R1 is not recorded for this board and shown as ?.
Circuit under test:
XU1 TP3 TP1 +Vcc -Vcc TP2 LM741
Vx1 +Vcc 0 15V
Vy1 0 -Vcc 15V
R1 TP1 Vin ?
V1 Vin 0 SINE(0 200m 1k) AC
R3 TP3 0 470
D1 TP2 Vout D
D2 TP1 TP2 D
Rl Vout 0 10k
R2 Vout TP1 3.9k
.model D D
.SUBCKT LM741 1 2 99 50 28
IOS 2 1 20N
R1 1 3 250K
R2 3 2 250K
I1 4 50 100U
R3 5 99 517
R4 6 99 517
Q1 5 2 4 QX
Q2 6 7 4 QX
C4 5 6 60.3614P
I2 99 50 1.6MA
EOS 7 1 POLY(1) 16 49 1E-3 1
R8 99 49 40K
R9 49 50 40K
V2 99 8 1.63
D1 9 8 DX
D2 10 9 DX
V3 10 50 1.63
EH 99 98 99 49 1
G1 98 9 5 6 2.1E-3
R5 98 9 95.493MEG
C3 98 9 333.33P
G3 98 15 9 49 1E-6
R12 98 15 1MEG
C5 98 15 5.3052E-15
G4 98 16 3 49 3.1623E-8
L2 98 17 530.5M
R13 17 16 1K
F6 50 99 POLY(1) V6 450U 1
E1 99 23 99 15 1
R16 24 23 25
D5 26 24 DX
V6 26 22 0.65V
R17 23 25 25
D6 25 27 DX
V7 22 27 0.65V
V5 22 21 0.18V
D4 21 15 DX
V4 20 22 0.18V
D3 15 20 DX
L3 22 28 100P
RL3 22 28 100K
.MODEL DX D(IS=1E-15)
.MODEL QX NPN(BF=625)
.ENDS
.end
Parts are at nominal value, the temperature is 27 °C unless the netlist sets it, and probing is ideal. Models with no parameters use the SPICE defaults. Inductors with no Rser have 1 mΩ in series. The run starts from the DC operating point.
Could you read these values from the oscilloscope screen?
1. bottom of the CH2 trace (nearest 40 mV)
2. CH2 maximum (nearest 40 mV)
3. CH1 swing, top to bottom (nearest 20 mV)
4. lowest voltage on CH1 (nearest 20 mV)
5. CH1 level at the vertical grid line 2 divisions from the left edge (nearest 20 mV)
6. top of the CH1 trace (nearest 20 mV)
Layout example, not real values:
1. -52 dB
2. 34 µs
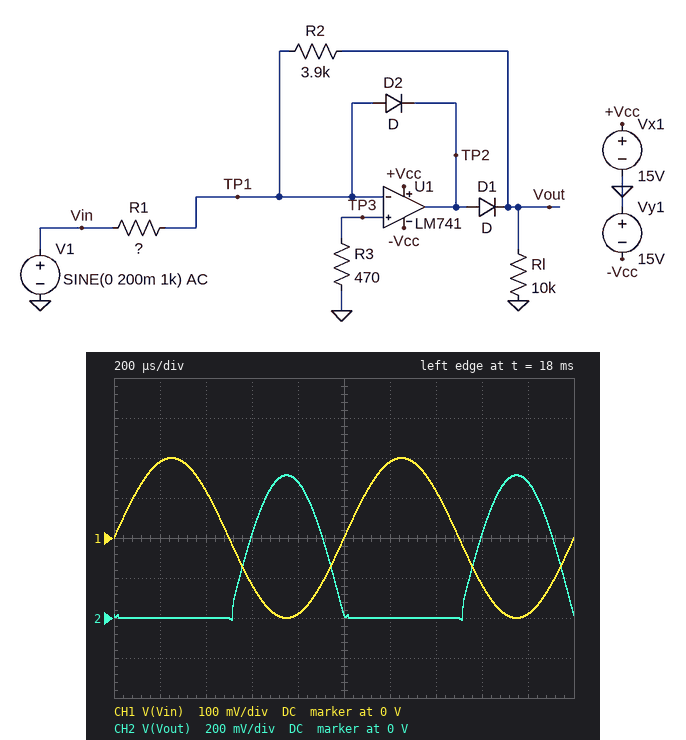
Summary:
1. 0 V
2. 720 mV
3. 400 mV
4. -200 mV
5. 120 mV
6. 200 mV
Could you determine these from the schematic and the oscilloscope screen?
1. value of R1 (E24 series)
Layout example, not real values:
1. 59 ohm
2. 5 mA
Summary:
1. 1.1 kΩ
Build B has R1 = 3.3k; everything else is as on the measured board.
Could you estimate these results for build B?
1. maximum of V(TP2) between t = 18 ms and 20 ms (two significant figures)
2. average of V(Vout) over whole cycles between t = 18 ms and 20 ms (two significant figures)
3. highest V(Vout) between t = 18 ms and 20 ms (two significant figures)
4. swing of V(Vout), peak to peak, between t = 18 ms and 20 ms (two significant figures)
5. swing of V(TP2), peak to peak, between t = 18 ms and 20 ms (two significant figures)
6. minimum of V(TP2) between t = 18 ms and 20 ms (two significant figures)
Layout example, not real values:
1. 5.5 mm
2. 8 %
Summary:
1. 830 mV
2. 77 mV
3. 240 mV
4. 250 mV
5. 1.4 V
6. -580 mV
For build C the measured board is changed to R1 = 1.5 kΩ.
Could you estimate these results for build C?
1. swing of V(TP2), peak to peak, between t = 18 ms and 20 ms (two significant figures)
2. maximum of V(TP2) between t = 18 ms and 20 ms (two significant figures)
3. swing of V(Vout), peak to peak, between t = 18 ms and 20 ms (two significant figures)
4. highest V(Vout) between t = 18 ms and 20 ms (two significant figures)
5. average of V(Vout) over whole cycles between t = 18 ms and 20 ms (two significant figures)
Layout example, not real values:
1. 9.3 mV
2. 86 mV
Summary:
1. 1.7 V
2. 1.1 V
3. 540 mV
4. 520 mV
5. 170 mV
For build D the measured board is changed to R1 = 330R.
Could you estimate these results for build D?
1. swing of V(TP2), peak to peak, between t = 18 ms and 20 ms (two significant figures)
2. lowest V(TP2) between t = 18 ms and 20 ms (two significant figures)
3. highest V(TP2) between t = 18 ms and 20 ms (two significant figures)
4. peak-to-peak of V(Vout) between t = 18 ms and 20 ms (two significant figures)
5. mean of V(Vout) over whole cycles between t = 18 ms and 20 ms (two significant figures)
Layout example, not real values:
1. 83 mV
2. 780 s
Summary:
1. 3.7 V
2. -640 mV
3. 3.0 V
4. 2.4 V
5. 760 mV
